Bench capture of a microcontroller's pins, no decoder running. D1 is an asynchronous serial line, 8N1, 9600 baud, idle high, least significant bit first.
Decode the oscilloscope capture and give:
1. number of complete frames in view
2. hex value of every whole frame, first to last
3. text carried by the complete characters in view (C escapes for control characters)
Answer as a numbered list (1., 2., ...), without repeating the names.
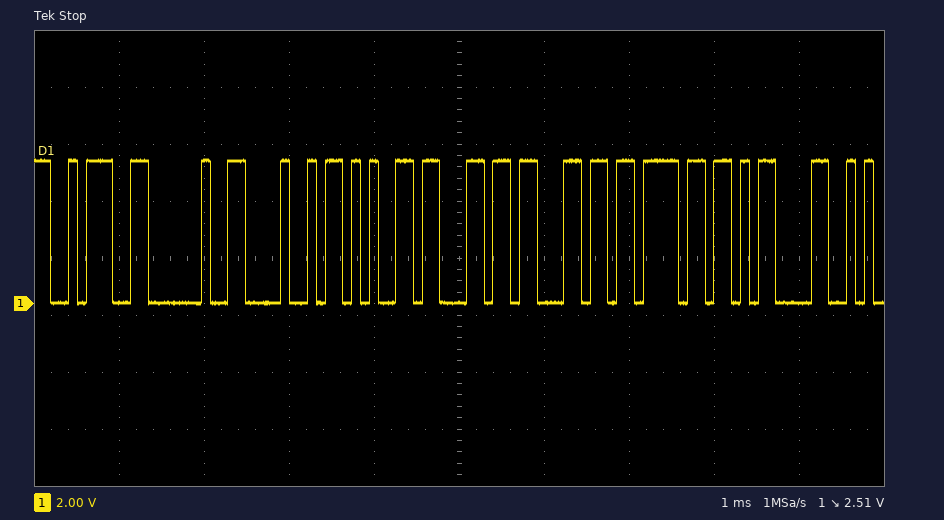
1. 8
2. 0x3A 0x20 0x48 0x65 0x6C 0x6C 0x6F 0x0D
3. ": Hello\r"
